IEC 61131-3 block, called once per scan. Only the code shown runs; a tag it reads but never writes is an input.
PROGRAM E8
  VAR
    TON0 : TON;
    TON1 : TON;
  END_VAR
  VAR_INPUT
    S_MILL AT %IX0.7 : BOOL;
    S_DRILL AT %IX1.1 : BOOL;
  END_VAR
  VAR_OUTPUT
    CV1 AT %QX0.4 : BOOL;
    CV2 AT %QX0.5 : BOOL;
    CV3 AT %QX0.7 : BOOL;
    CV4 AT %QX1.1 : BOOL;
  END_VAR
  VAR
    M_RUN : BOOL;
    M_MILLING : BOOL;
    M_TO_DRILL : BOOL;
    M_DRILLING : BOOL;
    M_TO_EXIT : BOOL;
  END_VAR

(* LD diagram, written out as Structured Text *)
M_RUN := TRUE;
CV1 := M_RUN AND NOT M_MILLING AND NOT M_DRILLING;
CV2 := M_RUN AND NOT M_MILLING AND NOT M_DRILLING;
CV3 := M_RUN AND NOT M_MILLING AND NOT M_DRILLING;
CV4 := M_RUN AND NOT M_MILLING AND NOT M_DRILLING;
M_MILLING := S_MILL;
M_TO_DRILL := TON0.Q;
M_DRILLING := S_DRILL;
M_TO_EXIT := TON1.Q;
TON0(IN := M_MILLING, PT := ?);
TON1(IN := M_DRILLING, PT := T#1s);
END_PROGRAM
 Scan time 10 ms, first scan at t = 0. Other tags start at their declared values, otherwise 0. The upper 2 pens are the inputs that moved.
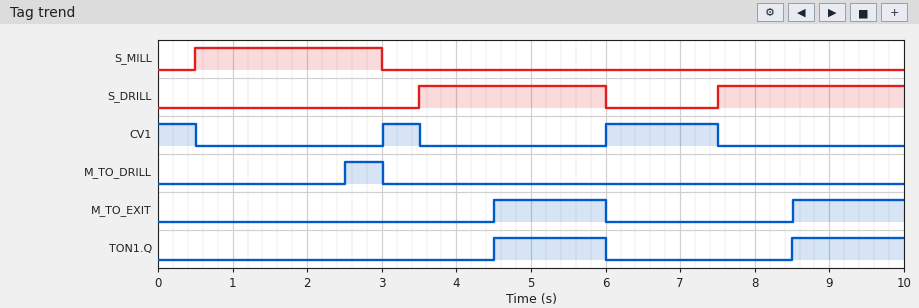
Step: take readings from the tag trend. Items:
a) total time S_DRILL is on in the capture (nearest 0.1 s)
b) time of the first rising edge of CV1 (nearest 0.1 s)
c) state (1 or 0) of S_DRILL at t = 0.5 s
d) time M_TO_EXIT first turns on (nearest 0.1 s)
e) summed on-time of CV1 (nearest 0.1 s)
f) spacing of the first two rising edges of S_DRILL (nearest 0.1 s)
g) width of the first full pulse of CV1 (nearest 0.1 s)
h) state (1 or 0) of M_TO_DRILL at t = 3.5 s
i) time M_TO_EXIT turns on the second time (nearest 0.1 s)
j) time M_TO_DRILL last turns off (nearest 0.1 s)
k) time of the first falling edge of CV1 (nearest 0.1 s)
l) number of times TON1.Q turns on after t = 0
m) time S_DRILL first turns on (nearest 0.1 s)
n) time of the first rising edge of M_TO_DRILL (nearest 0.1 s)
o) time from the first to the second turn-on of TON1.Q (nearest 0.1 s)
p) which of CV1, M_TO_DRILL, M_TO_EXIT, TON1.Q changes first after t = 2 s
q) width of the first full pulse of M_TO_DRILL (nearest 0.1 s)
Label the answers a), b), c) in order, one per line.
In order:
a) 5.0 s
b) 3.0 s
c) 0
d) 4.5 s
e) 2.5 s
f) 4.0 s
g) 0.5 s
h) 0
i) 8.5 s
j) 3.0 s
k) 0.5 s
l) 2
m) 3.5 s
n) 2.5 s
o) 4.0 s
p) M_TO_DRILL
q) 0.5 s
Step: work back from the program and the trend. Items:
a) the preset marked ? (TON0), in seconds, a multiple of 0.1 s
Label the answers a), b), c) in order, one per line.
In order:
a) 2.0 s
